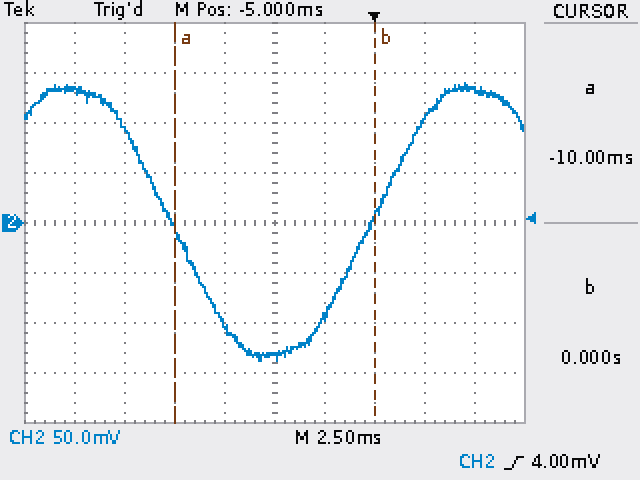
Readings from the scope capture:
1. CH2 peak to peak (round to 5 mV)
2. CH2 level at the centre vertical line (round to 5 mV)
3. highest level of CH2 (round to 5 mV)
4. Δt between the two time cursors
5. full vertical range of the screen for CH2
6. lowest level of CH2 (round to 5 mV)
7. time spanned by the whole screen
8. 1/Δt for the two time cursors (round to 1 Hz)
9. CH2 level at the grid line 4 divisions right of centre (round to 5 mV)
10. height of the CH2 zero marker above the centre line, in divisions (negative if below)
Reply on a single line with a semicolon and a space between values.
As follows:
280 mV; -135 mV; 140 mV; 10.00 ms; 400 mV; -140 mV; 25 ms; 100 Hz; 135 mV; 0.0 div
